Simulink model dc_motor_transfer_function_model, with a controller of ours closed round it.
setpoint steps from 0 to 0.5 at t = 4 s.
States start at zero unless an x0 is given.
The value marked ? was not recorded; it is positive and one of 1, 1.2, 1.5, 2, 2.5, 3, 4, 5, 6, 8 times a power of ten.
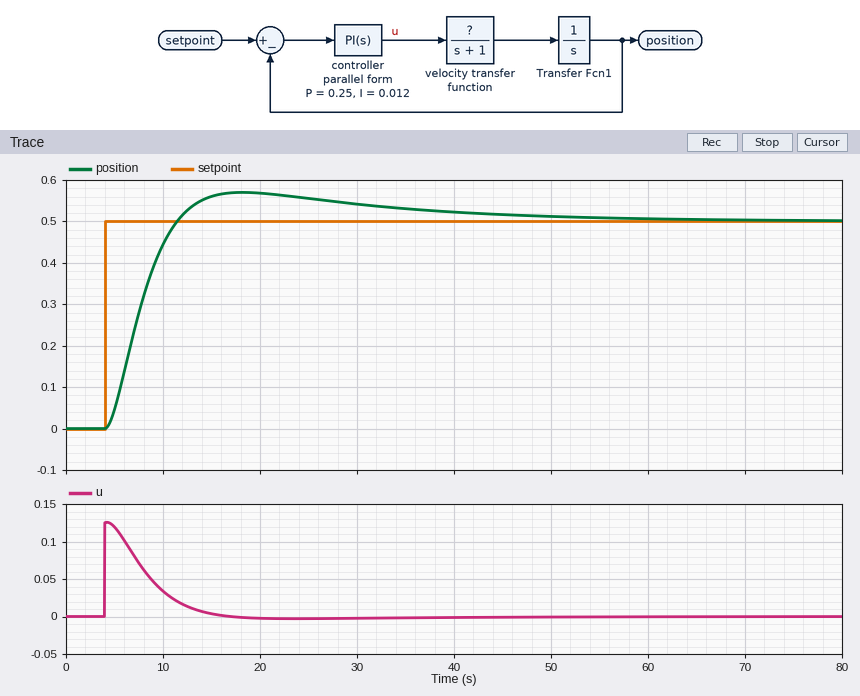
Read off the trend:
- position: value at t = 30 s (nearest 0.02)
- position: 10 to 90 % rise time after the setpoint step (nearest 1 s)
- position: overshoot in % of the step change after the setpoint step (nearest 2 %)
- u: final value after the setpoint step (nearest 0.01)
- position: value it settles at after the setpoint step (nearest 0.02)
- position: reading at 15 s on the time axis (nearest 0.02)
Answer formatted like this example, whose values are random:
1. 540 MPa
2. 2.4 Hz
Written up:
1. 0.54
2. 5 s
3. 14 %
4. 0.00
5. 0.50
6. 0.56
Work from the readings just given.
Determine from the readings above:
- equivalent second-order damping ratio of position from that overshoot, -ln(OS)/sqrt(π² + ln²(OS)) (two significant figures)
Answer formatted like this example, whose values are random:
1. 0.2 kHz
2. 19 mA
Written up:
1. 0.53
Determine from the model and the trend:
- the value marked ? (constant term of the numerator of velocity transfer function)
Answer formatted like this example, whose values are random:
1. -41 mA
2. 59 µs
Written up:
1. 1
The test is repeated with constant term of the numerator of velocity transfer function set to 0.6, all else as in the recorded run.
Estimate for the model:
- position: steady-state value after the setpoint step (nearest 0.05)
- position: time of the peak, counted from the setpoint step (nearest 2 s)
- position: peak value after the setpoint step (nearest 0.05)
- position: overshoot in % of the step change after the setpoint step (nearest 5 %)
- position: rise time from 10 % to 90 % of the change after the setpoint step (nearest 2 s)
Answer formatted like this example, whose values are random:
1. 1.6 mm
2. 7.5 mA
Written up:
1. 0.50
2. 22 s
3. 0.60
4. 20 %
5. 8 s
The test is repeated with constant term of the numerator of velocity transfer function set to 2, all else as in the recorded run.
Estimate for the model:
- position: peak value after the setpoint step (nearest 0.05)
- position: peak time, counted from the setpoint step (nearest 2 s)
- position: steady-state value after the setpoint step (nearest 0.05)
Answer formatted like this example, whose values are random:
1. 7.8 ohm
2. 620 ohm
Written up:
1. 0.55
2. 6 s
3. 0.50
